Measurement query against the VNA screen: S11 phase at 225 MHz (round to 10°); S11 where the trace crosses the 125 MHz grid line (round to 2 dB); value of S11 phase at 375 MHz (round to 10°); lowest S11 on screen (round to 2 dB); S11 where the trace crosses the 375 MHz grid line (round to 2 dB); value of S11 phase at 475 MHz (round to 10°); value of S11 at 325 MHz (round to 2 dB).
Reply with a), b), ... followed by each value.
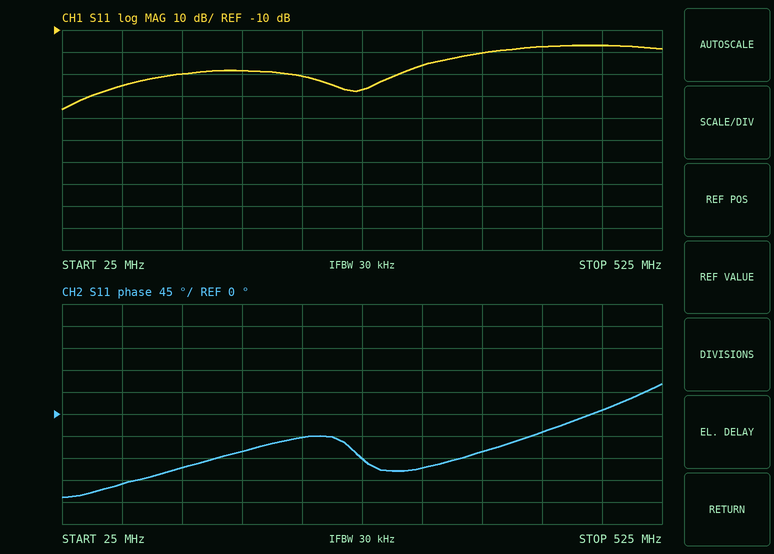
a) -50°
b) -30 dB
c) -80°
d) -46 dB
e) -20 dB
f) 10°
g) -26 dB
